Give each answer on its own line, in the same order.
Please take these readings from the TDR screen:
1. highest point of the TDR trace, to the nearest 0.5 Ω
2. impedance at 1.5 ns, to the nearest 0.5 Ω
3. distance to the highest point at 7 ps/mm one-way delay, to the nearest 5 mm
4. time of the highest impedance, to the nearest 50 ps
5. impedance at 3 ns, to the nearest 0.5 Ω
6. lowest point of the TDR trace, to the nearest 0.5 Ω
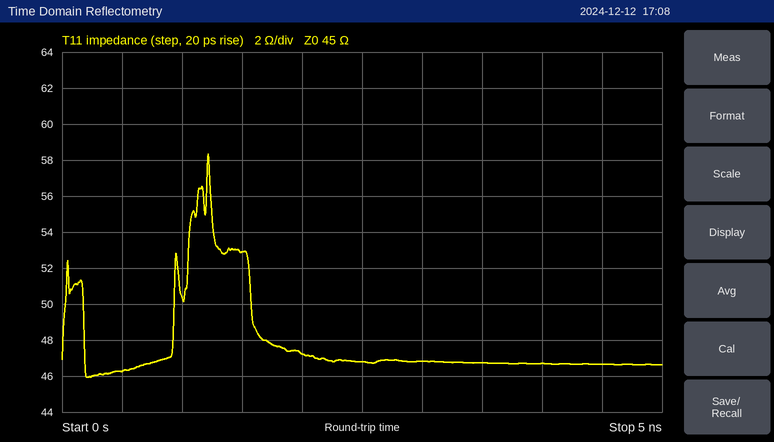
58.5 Ω
53.0 Ω
85 mm
1.20 ns
47.0 Ω
46.0 Ω
